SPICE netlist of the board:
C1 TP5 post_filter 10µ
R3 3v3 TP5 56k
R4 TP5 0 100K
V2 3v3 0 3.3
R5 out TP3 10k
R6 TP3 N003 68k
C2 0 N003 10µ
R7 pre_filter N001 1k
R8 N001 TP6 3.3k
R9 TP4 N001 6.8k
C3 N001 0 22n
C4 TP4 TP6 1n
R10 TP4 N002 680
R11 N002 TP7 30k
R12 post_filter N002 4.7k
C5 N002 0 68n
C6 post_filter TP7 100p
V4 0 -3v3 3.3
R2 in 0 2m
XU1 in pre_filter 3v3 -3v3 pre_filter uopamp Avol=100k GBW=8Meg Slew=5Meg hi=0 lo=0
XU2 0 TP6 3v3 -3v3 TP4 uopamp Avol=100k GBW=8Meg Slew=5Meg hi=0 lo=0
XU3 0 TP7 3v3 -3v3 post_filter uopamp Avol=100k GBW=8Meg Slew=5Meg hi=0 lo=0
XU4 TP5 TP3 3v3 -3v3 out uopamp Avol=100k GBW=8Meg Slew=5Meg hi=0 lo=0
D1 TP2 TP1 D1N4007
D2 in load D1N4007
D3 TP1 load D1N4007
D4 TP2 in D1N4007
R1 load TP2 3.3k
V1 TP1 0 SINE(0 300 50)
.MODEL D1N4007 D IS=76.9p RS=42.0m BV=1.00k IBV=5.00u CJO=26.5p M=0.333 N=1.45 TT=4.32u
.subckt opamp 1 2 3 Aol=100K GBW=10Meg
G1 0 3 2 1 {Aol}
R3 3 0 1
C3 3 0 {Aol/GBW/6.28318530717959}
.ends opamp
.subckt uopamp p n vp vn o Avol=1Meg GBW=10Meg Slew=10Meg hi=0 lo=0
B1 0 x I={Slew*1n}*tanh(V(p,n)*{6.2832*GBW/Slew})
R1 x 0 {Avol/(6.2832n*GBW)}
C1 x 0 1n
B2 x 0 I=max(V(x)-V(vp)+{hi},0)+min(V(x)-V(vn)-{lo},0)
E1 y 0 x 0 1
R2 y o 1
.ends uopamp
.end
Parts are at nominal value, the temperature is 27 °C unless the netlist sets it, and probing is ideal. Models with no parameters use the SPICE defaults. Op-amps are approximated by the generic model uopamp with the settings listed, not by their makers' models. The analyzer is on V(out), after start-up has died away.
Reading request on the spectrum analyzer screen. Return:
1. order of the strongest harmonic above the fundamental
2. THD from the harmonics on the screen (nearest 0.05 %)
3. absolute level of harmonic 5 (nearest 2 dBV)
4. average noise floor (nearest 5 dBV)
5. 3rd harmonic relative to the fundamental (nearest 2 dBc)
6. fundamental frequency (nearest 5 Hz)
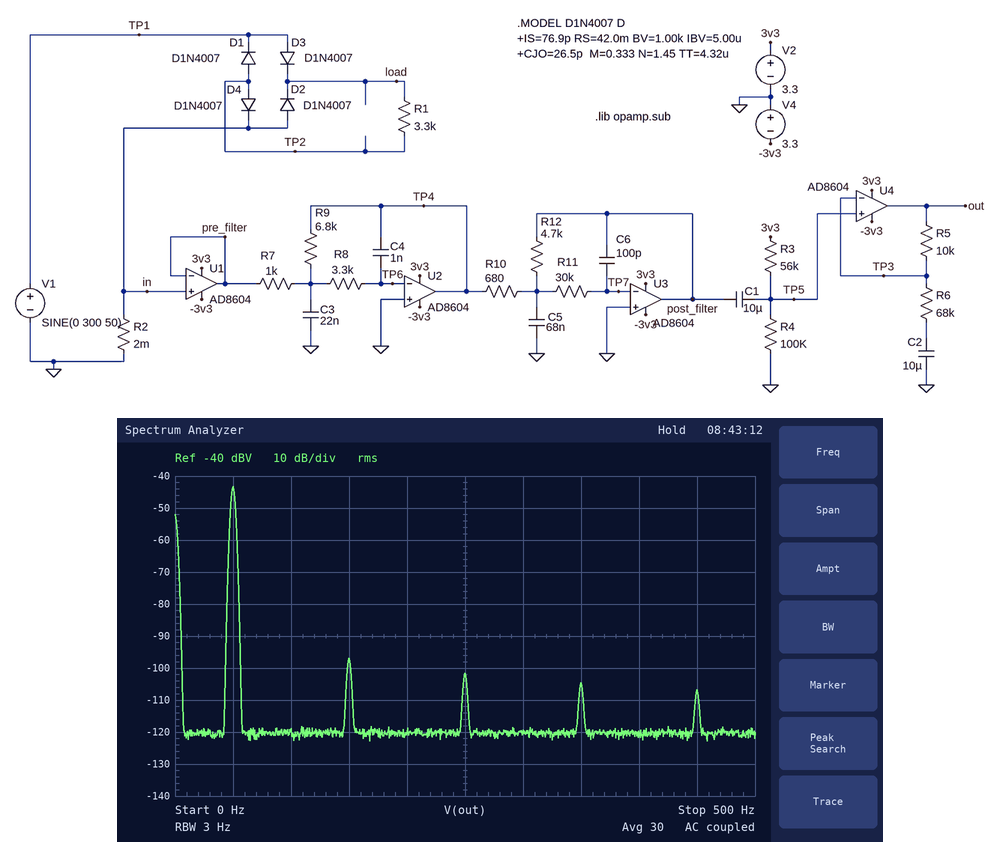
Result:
3
0.25 %
-102 dBV
-120 dBV
-54 dBc
50 Hz
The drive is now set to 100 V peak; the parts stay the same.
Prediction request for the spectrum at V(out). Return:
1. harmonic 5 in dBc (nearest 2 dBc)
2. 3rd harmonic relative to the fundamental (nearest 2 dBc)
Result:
-50 dBc
-44 dBc
